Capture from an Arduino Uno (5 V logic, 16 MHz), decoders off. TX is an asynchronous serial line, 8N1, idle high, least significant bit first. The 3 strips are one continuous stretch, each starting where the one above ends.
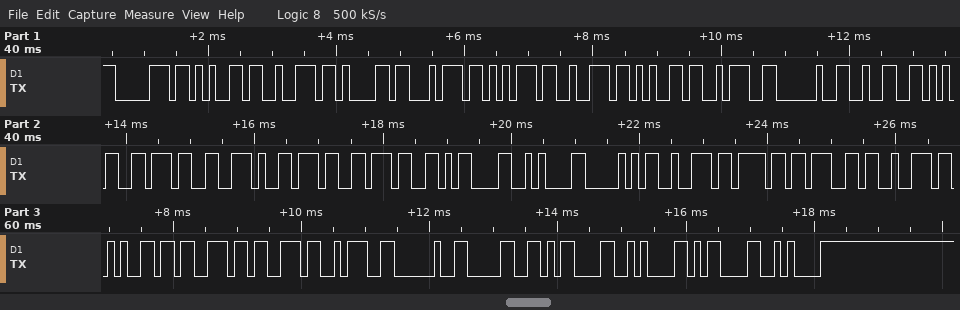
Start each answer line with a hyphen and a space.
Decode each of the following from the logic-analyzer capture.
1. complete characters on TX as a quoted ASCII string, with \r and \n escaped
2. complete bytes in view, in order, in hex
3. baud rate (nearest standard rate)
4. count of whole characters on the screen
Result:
- "perature: 257.77\r\nProgress: 0\r\n\r\n"
- 70 65 72 61 74 75 72 65 3A 20 32 35 37 2E 37 37 0D 0A 50 72 6F 67 72 65 73 73 3A 20 30 0D 0A 0D 0A
- 9600 baud
- 33
